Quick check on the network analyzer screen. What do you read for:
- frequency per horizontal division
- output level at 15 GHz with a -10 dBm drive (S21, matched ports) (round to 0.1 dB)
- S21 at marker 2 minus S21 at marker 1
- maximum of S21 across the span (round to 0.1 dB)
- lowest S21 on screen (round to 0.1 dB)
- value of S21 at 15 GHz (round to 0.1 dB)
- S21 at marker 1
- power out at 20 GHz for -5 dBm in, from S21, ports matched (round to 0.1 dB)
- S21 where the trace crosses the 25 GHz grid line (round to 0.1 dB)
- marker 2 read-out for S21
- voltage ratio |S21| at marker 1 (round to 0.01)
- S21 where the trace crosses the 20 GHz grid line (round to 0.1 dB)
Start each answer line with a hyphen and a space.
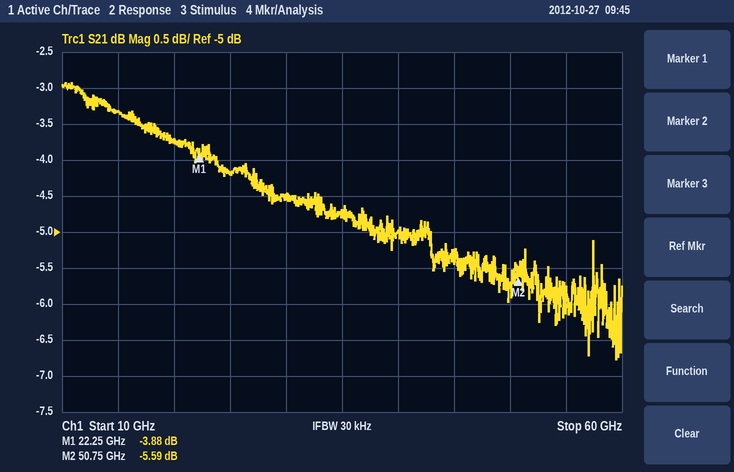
- 5 GHz
- -13.3 dBm
- -1.71 dB
- -2.9 dB
- -6.8 dB
- -3.3 dB
- -3.88 dB
- -8.7 dBm
- -4.2 dB
- -5.59 dB
- 0.64
- -3.7 dB
